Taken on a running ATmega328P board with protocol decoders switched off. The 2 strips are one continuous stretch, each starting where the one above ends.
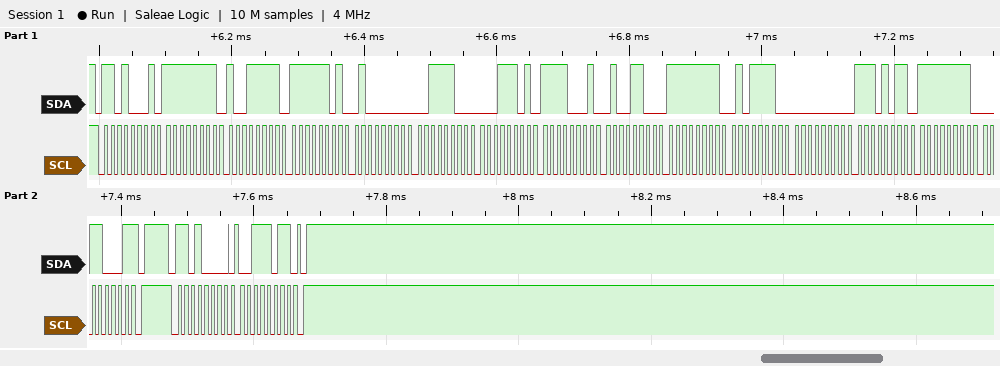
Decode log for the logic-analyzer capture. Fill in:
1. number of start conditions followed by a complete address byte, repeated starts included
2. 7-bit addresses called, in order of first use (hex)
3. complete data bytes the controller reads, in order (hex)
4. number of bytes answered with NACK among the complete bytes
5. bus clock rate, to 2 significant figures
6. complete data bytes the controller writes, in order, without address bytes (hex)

2
0x68
FF 9F FD 40 3C 1D F1 4C FF 5E 00 EB FF 31
1
100 kHz
3B
